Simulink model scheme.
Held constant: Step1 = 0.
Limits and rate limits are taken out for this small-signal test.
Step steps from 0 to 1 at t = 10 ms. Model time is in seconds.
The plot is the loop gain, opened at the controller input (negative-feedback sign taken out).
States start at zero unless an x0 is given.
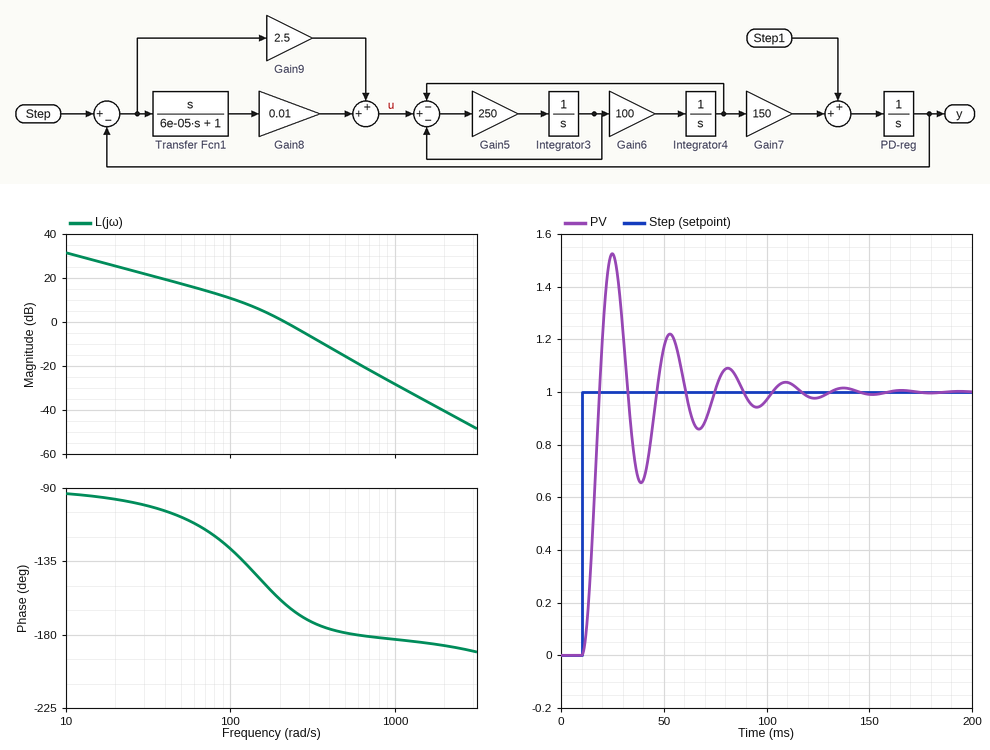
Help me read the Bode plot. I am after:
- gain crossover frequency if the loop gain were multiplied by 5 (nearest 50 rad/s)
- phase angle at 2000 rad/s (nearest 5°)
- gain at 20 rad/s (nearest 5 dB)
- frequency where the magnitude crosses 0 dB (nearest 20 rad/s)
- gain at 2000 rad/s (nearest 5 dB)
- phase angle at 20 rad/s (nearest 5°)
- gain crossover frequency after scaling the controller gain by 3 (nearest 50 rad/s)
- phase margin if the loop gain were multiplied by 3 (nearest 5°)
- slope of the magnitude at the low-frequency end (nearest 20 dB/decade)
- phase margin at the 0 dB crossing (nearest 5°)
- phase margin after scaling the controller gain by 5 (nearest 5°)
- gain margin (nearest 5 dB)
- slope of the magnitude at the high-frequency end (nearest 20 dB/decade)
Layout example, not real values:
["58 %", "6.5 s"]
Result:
["450 rad/s", "-185°", "25 dB", "220 rad/s", "-40 dB", "-95°", "350 rad/s", "5°", "-20 dB/decade", "20°", "0°", "20 dB", "-40 dB/decade"]
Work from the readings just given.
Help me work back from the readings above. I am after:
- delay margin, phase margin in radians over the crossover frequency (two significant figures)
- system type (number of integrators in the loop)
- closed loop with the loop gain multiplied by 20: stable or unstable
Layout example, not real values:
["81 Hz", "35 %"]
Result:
["0.0016 s", "1", "unstable"]
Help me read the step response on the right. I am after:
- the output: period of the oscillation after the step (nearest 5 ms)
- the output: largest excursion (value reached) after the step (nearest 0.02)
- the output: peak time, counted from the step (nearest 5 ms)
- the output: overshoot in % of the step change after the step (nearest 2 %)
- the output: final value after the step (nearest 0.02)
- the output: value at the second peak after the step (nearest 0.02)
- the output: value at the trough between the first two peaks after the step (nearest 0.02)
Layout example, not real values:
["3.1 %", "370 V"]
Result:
["30 ms", "1.52", "15 ms", "52 %", "1.00", "1.22", "0.66"]
